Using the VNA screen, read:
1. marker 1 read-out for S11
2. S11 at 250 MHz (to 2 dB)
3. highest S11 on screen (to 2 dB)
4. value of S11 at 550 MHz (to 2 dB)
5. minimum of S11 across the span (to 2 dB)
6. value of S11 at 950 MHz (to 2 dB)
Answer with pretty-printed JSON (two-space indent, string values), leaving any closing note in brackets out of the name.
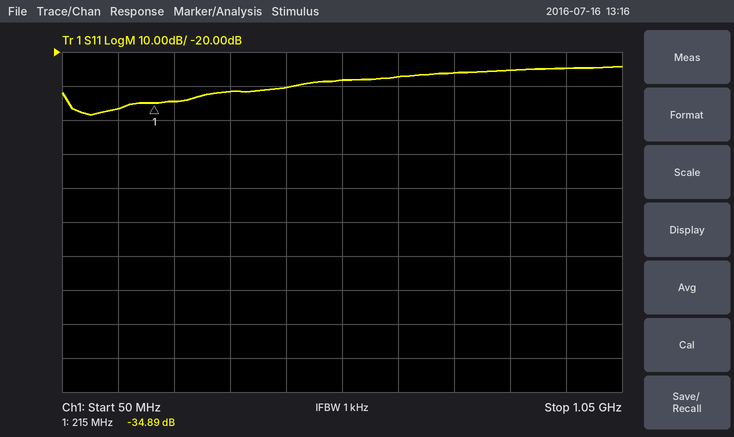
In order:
{
  "marker 1 read-out for S11": "-34.89 dB",
  "S11 at 250 MHz": "-34 dB",
  "highest S11 on screen": "-24 dB",
  "value of S11 at 550 MHz": "-28 dB",
  "minimum of S11 across the span": "-38 dB",
  "value of S11 at 950 MHz": "-24 dB"
}
